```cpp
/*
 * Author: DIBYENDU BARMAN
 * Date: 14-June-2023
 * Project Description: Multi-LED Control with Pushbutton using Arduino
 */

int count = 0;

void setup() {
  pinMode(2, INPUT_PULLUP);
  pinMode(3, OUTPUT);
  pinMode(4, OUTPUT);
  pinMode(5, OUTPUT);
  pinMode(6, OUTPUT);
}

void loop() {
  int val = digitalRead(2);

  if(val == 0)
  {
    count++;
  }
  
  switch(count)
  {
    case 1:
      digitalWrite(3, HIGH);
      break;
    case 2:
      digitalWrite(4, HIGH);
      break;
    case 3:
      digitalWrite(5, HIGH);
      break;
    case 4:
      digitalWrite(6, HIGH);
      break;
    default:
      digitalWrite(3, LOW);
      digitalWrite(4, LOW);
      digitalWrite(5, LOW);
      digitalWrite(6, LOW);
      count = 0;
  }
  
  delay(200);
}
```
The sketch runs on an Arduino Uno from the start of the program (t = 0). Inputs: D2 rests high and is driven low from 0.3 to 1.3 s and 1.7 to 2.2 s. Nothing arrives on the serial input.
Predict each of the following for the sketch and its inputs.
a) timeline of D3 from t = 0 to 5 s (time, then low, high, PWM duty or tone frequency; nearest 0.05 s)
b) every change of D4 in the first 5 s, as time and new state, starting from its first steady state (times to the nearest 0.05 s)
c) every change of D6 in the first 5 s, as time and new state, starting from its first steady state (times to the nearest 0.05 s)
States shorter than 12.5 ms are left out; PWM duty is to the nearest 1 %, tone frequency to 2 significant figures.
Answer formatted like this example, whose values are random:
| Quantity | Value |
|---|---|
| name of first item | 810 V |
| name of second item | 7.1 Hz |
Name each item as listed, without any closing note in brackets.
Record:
| Quantity | Value |
|---|---|
| timeline of D3 from t = 0 to 5 s | 0 s low; 0.4 s high; 1.2 s low; 1.8 s high |
| every change of D4 in the first 5 s, as time and new state, starting from its first steady state | 0 s low; 0.6 s high; 1.2 s low; 2 s high |
| every change of D6 in the first 5 s, as time and new state, starting from its first steady state | 0 s low; 1 s high; 1.2 s low |
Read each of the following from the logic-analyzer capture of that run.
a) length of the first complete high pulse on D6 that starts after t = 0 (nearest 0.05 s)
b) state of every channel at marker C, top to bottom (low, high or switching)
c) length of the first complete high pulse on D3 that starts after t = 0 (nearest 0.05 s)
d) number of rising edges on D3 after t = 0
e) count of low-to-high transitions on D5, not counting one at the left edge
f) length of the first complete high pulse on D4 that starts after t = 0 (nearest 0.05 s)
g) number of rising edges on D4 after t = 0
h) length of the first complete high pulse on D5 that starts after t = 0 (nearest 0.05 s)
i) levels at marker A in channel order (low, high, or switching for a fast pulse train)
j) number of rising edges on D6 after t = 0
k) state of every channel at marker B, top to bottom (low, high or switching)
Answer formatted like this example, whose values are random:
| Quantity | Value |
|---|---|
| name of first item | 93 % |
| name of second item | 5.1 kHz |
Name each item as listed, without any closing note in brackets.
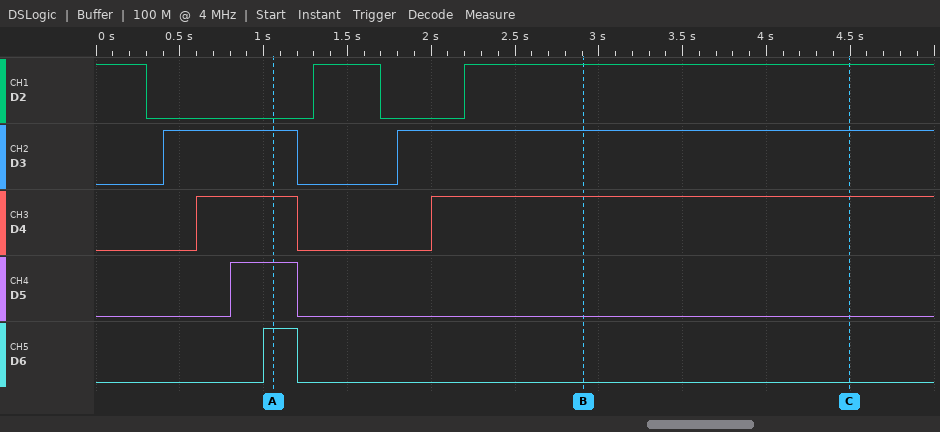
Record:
| Quantity | Value |
|---|---|
| length of the first complete high pulse on D6 that starts after t = 0 | 0.20 s |
| state of every channel at marker C, top to bottom | D2 high, D3 high, D4 high, D5 low, D6 low |
| length of the first complete high pulse on D3 that starts after t = 0 | 0.80 s |
| number of rising edges on D3 after t = 0 | 2 |
| count of low-to-high transitions on D5, not counting one at the left edge | 1 |
| length of the first complete high pulse on D4 that starts after t = 0 | 0.60 s |
| number of rising edges on D4 after t = 0 | 2 |
| length of the first complete high pulse on D5 that starts after t = 0 | 0.40 s |
| levels at marker A in channel order | D2 low, D3 high, D4 high, D5 high, D6 high |
| number of rising edges on D6 after t = 0 | 1 |
| state of every channel at marker B, top to bottom | D2 high, D3 high, D4 high, D5 low, D6 low |
